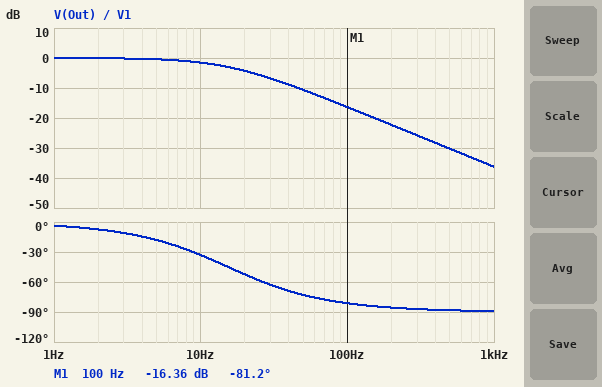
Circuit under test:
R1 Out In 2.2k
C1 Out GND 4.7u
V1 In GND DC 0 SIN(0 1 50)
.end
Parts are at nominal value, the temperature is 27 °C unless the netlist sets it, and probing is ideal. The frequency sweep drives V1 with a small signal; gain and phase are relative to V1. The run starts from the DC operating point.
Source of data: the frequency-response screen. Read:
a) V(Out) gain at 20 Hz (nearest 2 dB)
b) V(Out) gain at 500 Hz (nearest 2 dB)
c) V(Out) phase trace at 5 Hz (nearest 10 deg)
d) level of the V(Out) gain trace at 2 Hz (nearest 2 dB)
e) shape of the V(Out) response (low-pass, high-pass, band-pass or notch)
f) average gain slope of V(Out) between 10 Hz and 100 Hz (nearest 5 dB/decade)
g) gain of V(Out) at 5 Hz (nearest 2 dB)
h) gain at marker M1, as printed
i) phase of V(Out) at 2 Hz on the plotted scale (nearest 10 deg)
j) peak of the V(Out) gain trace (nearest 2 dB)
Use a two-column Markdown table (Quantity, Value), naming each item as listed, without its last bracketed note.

| Quantity | Value |
|---|---|
| V(Out) gain at 20 Hz | -4 dB |
| V(Out) gain at 500 Hz | -30 dB |
| V(Out) phase trace at 5 Hz | -20 deg |
| level of the V(Out) gain trace at 2 Hz | 0 dB |
| shape of the V(Out) response | low-pass |
| average gain slope of V(Out) between 10 Hz and 100 Hz | -15 dB/decade |
| gain of V(Out) at 5 Hz | 0 dB |
| gain at marker M1, as printed | -16.36 dB |
| phase of V(Out) at 2 Hz on the plotted scale | -10 deg |
| peak of the V(Out) gain trace | 0 dB |
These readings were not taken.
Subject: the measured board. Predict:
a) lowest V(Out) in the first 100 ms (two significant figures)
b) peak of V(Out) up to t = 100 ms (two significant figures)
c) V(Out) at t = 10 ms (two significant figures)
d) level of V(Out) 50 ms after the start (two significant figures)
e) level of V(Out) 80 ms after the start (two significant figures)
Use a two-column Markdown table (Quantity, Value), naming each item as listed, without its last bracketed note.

| Quantity | Value |
|---|---|
| lowest V(Out) in the first 100 ms | -290 mV |
| peak of V(Out) up to t = 100 ms | 410 mV |
| V(Out) at t = 10 ms | 390 mV |
| level of V(Out) 50 ms after the start | 280 mV |
| level of V(Out) 80 ms after the start | -280 mV |
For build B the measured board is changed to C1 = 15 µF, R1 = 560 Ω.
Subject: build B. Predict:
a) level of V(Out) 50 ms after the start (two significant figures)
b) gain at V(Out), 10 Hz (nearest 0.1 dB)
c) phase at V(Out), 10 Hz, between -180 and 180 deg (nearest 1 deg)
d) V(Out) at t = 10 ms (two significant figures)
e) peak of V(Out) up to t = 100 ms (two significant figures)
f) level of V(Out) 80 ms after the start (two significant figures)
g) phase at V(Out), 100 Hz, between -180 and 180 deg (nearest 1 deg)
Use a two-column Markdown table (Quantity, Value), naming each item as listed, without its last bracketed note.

| Quantity | Value |
|---|---|
| level of V(Out) 50 ms after the start | 330 mV |
| gain at V(Out), 10 Hz | -1.1 dB |
| phase at V(Out), 10 Hz, between -180 and 180 deg | -28 deg |
| V(Out) at t = 10 ms | 430 mV |
| peak of V(Out) up to t = 100 ms | 470 mV |
| level of V(Out) 80 ms after the start | -330 mV |
| phase at V(Out), 100 Hz, between -180 and 180 deg | -79 deg |
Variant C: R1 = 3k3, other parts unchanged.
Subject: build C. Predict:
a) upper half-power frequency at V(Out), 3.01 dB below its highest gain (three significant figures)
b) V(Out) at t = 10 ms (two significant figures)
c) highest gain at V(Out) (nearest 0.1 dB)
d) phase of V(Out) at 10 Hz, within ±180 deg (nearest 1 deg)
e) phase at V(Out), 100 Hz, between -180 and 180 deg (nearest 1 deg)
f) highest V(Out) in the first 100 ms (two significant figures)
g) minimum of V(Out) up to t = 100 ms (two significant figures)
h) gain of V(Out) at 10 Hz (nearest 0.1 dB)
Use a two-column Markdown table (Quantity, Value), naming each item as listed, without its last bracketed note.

| Quantity | Value |
|---|---|
| upper half-power frequency at V(Out), 3.01 dB below its highest gain | 10.3 Hz |
| V(Out) at t = 10 ms | 300 mV |
| highest gain at V(Out) | 0 dB |
| phase of V(Out) at 10 Hz, within ±180 deg | -44 deg |
| phase at V(Out), 100 Hz, between -180 and 180 deg | -84 deg |
| highest V(Out) in the first 100 ms | 310 mV |
| minimum of V(Out) up to t = 100 ms | -200 mV |
| gain of V(Out) at 10 Hz | -2.9 dB |
